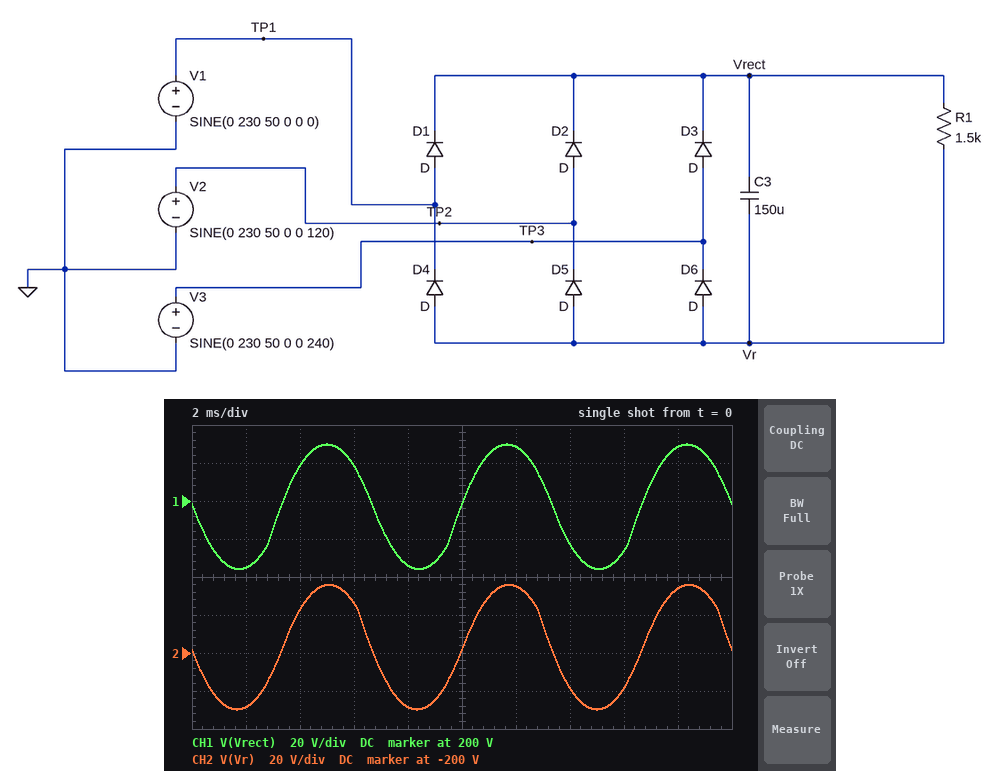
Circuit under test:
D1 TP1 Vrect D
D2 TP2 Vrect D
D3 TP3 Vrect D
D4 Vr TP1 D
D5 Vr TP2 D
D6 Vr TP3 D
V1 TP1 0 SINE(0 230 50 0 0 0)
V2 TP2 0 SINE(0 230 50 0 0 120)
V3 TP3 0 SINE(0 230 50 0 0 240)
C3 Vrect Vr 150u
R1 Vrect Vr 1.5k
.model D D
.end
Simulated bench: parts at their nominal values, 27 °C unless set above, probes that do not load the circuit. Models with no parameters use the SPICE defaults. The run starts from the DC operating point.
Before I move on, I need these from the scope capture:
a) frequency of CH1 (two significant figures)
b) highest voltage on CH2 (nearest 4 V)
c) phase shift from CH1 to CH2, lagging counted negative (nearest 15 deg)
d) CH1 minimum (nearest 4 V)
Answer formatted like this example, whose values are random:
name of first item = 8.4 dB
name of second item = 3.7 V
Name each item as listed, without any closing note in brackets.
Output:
frequency of CH1 = 150 Hz
highest voltage on CH2 = -164 V
phase shift from CH1 to CH2, lagging counted negative = 0 deg
CH1 minimum = 164 V
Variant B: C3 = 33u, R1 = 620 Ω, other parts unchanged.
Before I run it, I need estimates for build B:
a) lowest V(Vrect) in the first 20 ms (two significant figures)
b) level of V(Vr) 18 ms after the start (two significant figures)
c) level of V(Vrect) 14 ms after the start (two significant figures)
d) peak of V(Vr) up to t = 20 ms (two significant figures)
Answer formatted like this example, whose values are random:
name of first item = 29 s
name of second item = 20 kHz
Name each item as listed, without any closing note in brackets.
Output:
lowest V(Vrect) in the first 20 ms = 140 V
level of V(Vr) 18 ms after the start = -150 V
level of V(Vrect) 14 ms after the start = 170 V
peak of V(Vr) up to t = 20 ms = -140 V
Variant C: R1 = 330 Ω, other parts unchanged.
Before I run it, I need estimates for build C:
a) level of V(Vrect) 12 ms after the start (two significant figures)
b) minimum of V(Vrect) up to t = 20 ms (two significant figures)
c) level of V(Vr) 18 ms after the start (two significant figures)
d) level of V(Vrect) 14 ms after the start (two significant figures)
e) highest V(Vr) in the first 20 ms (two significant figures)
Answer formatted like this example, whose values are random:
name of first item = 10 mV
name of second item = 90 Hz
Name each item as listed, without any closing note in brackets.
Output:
level of V(Vrect) 12 ms after the start = 230 V
minimum of V(Vrect) up to t = 20 ms = 150 V
level of V(Vr) 18 ms after the start = -160 V
level of V(Vrect) 14 ms after the start = 170 V
highest V(Vr) in the first 20 ms = -150 V
